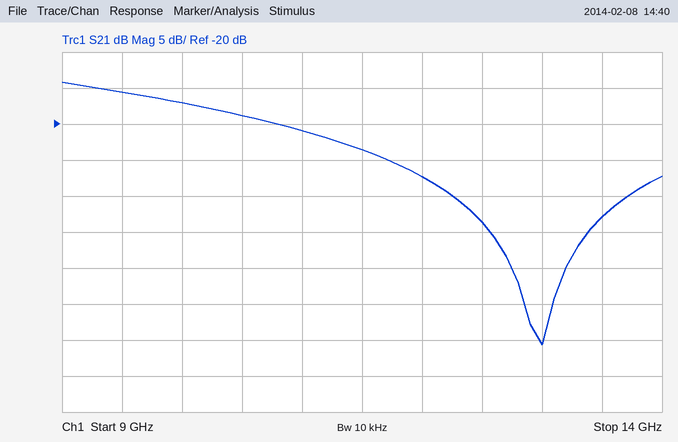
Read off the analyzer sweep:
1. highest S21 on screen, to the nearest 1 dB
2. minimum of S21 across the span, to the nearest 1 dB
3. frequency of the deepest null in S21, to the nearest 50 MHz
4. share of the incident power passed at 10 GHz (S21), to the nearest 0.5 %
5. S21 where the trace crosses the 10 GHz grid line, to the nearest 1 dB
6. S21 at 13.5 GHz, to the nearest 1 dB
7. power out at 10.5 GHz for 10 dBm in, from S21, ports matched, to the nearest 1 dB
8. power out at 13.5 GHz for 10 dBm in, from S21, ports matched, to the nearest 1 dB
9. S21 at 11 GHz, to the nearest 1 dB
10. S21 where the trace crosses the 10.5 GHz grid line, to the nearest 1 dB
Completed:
-14 dB
-51 dB
13.00 GHz
2.0 %
-17 dB
-33 dB
-9 dBm
-23 dBm
-21 dB
-19 dB
